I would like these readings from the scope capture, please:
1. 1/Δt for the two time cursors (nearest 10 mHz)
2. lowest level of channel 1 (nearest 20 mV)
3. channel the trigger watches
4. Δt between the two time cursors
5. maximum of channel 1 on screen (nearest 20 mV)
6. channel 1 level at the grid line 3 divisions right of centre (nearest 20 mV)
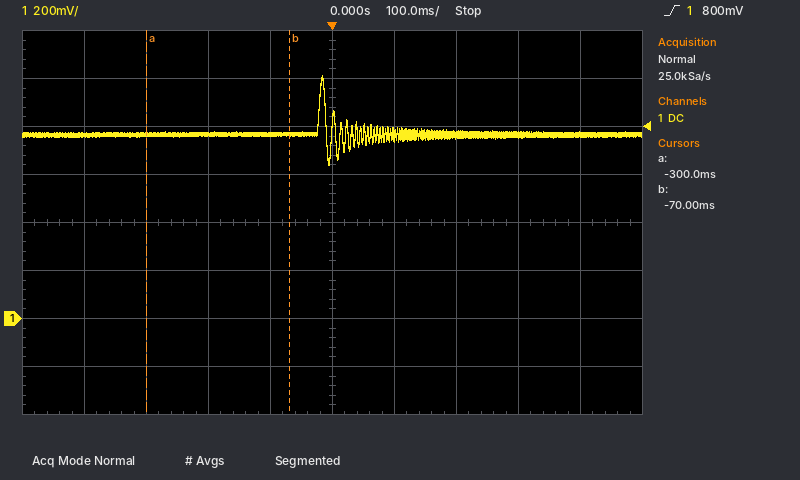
4.35 Hz
640 mV
channel 1
230 ms
1.02 V
760 mV
